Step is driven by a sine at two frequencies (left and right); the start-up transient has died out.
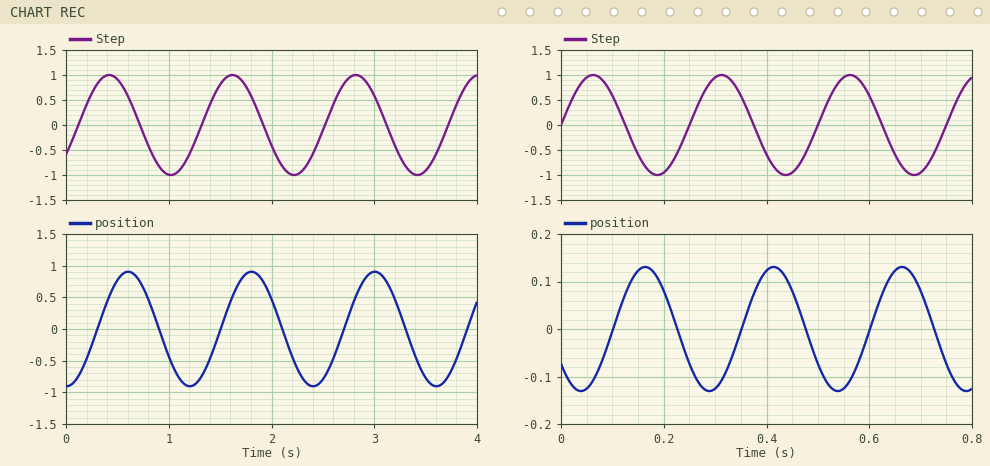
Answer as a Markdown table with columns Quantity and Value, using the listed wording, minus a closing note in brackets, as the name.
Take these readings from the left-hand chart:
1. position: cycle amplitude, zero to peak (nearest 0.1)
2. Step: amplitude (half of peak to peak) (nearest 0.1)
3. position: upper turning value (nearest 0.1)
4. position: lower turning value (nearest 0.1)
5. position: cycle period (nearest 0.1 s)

| Quantity | Value |
|---|---|
| position: cycle amplitude, zero to peak | 0.9 |
| Step: amplitude (half of peak to peak) | 1.0 |
| position: upper turning value | 0.9 |
| position: lower turning value | -0.9 |
| position: cycle period | 1.2 s |
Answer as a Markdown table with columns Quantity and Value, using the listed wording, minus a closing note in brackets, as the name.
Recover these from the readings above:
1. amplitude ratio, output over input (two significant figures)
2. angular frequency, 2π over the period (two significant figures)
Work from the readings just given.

| Quantity | Value |
|---|---|
| amplitude ratio, output over input | 0.90 |
| angular frequency, 2π over the period | 5.2 rad/s |
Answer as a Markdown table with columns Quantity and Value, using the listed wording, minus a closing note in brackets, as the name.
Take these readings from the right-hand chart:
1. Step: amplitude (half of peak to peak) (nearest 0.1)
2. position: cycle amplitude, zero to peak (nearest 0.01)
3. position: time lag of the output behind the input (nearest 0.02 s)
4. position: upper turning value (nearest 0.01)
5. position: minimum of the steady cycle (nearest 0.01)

| Quantity | Value |
|---|---|
| Step: amplitude (half of peak to peak) | 1.0 |
| position: cycle amplitude, zero to peak | 0.13 |
| position: time lag of the output behind the input | 0.10 s |
| position: upper turning value | 0.13 |
| position: minimum of the steady cycle | -0.13 |
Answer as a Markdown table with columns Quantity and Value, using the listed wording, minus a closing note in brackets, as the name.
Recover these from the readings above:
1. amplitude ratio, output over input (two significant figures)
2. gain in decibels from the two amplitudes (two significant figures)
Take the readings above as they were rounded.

| Quantity | Value |
|---|---|
| amplitude ratio, output over input | 0.13 |
| gain in decibels from the two amplitudes | -18 dB |
